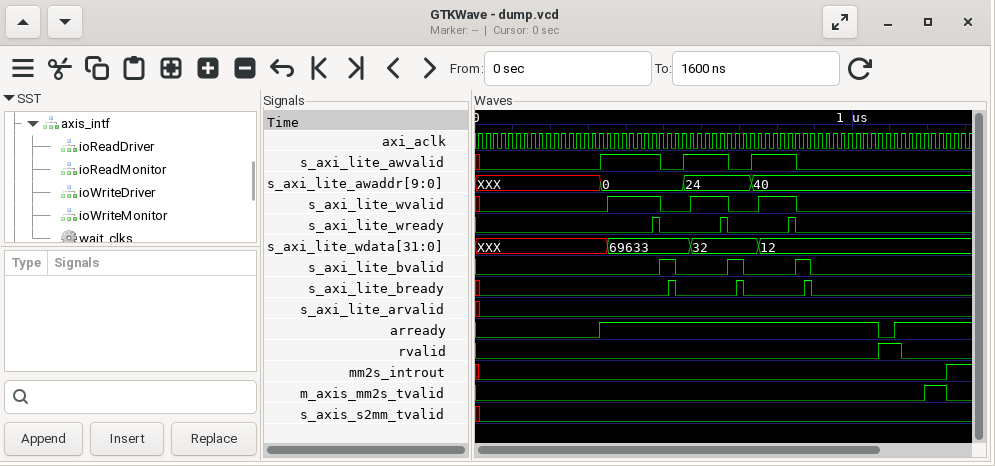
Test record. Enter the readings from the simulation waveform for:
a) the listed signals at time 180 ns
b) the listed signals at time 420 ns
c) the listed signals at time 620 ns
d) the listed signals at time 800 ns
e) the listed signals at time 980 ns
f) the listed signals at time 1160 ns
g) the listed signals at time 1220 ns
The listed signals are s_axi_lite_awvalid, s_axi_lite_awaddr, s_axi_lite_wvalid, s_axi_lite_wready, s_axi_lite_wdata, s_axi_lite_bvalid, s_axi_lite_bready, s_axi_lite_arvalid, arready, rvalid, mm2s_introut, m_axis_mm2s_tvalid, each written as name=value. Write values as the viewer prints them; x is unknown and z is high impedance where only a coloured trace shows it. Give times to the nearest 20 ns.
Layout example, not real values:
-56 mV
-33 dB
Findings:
s_axi_lite_awvalid=0, s_axi_lite_awaddr=XXX, s_axi_lite_wvalid=0, s_axi_lite_wready=0, s_axi_lite_wdata=XXX, s_axi_lite_bvalid=0, s_axi_lite_bready=0, s_axi_lite_arvalid=0, arready=0, rvalid=0, mm2s_introut=0, m_axis_mm2s_tvalid=0
s_axi_lite_awvalid=1, s_axi_lite_awaddr=0, s_axi_lite_wvalid=1, s_axi_lite_wready=0, s_axi_lite_wdata=69633, s_axi_lite_bvalid=0, s_axi_lite_bready=0, s_axi_lite_arvalid=0, arready=1, rvalid=0, mm2s_introut=0, m_axis_mm2s_tvalid=0
s_axi_lite_awvalid=1, s_axi_lite_awaddr=24, s_axi_lite_wvalid=1, s_axi_lite_wready=0, s_axi_lite_wdata=32, s_axi_lite_bvalid=0, s_axi_lite_bready=0, s_axi_lite_arvalid=0, arready=1, rvalid=0, mm2s_introut=0, m_axis_mm2s_tvalid=0
s_axi_lite_awvalid=1, s_axi_lite_awaddr=40, s_axi_lite_wvalid=1, s_axi_lite_wready=0, s_axi_lite_wdata=12, s_axi_lite_bvalid=0, s_axi_lite_bready=0, s_axi_lite_arvalid=0, arready=1, rvalid=0, mm2s_introut=0, m_axis_mm2s_tvalid=0
s_axi_lite_awvalid=0, s_axi_lite_awaddr=40, s_axi_lite_wvalid=0, s_axi_lite_wready=0, s_axi_lite_wdata=12, s_axi_lite_bvalid=0, s_axi_lite_bready=0, s_axi_lite_arvalid=0, arready=1, rvalid=0, mm2s_introut=0, m_axis_mm2s_tvalid=0
s_axi_lite_awvalid=0, s_axi_lite_awaddr=40, s_axi_lite_wvalid=0, s_axi_lite_wready=0, s_axi_lite_wdata=12, s_axi_lite_bvalid=0, s_axi_lite_bready=0, s_axi_lite_arvalid=0, arready=1, rvalid=0, mm2s_introut=0, m_axis_mm2s_tvalid=0
s_axi_lite_awvalid=0, s_axi_lite_awaddr=40, s_axi_lite_wvalid=0, s_axi_lite_wready=0, s_axi_lite_wdata=12, s_axi_lite_bvalid=0, s_axi_lite_bready=0, s_axi_lite_arvalid=0, arready=1, rvalid=0, mm2s_introut=0, m_axis_mm2s_tvalid=1
